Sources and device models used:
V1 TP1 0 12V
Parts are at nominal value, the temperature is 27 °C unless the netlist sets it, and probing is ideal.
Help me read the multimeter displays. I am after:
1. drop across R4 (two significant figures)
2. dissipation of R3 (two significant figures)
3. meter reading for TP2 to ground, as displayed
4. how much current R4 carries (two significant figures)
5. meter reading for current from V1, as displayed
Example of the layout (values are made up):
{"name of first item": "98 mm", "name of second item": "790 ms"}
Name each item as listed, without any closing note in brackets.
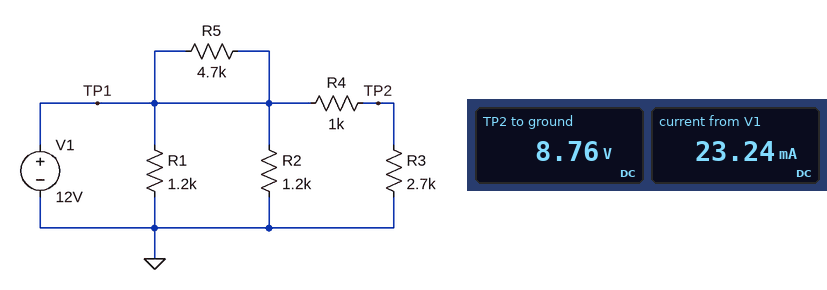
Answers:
{"drop across R4": "3.2 V", "dissipation of R3": "28 mW", "meter reading for TP2 to ground, as displayed": "8.76 V", "how much current R4 carries": "3.2 mA", "meter reading for current from V1, as displayed": "23.24 mA"}
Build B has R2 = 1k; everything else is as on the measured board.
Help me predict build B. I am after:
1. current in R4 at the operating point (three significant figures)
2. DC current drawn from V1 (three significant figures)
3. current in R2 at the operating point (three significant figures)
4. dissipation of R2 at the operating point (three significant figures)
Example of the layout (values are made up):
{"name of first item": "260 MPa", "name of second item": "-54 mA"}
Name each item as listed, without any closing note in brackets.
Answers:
{"current in R4 at the operating point": "3.24 mA", "DC current drawn from V1": "25.2 mA", "current in R2 at the operating point": "12.0 mA", "dissipation of R2 at the operating point": "144 mW"}
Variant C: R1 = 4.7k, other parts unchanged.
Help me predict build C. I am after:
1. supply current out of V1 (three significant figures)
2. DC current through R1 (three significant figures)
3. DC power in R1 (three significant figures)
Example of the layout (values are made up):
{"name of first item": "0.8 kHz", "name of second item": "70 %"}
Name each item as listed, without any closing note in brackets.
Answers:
{"supply current out of V1": "15.8 mA", "DC current through R1": "2.55 mA", "DC power in R1": "30.6 mW"}
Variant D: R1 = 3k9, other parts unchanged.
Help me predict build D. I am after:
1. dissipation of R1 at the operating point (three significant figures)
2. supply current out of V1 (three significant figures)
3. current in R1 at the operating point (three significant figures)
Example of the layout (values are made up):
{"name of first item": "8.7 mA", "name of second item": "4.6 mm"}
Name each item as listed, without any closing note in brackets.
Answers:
{"dissipation of R1 at the operating point": "36.9 mW", "supply current out of V1": "16.3 mA", "current in R1 at the operating point": "3.08 mA"}
